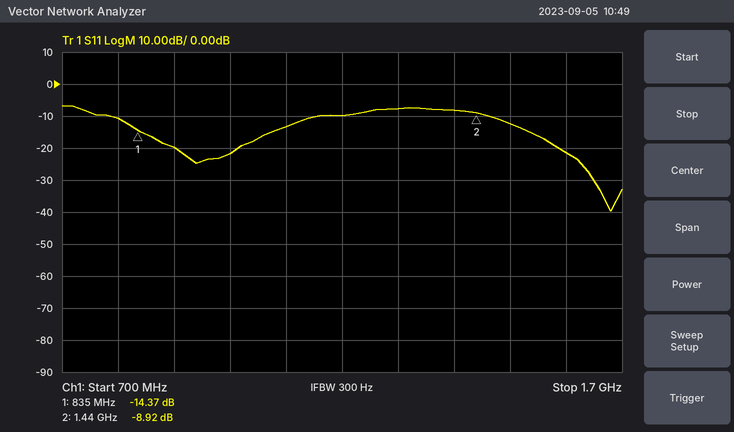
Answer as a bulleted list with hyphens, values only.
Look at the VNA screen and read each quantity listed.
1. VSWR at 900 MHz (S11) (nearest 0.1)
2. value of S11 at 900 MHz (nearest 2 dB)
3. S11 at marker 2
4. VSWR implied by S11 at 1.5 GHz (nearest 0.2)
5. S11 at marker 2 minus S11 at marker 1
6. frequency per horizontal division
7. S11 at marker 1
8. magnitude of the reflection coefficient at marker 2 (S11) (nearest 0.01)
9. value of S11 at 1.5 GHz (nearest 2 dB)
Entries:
- 1.2
- -20 dB
- -8.92 dB
- 1.6
- 5.45 dB
- 100 MHz
- -14.37 dB
- 0.36
- -12 dB
